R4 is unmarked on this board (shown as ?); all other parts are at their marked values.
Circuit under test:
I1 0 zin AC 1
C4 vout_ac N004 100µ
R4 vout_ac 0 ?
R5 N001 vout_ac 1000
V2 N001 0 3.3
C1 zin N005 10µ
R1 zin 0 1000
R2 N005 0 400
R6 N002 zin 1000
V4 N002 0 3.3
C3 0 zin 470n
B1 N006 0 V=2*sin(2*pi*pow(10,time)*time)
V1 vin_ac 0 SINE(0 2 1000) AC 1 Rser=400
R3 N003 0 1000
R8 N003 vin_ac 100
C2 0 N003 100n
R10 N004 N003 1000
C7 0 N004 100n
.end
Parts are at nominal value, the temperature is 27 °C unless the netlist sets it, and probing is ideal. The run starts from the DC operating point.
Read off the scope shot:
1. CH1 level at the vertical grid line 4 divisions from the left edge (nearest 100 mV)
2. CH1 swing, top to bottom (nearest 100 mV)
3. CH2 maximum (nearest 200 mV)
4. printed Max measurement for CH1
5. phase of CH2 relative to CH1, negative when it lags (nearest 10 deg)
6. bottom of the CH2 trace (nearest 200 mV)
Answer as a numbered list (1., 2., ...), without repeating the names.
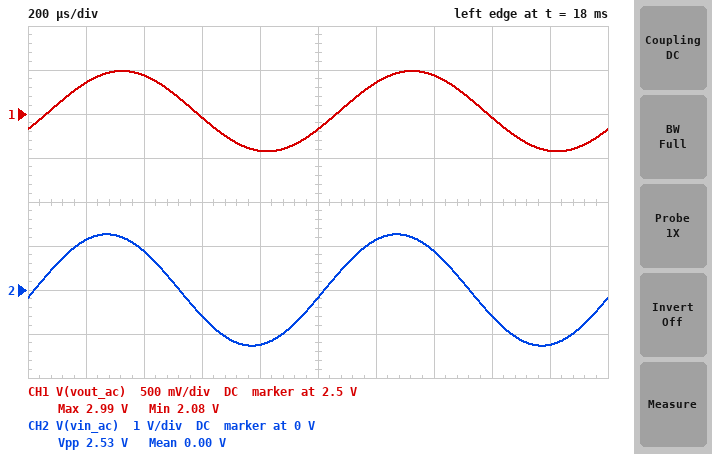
1. 2.1 V
2. 900 mV
3. 1.2 V
4. 2.99 V
5. 20 deg
6. -1.2 V
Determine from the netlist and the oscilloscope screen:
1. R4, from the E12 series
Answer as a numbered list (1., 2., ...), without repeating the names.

1. 3.3 kΩ
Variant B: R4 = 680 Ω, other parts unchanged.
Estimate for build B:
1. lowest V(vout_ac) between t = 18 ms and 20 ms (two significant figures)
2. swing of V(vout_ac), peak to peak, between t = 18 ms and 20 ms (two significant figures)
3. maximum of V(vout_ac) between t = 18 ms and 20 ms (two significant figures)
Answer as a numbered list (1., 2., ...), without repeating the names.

1. 1.0 V
2. 600 mV
3. 1.6 V
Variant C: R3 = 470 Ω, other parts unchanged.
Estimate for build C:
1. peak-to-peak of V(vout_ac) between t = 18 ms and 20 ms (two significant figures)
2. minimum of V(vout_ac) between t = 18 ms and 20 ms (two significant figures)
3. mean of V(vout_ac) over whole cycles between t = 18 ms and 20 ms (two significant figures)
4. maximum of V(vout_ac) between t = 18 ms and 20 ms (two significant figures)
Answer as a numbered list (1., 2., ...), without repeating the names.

1. 700 mV
2. 2.2 V
3. 2.5 V
4. 2.9 V
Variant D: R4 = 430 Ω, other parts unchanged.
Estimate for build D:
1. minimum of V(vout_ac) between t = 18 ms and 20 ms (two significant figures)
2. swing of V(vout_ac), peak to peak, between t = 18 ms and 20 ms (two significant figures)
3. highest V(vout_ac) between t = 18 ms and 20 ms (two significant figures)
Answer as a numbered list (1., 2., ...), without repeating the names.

1. 750 mV
2. 480 mV
3. 1.2 V
